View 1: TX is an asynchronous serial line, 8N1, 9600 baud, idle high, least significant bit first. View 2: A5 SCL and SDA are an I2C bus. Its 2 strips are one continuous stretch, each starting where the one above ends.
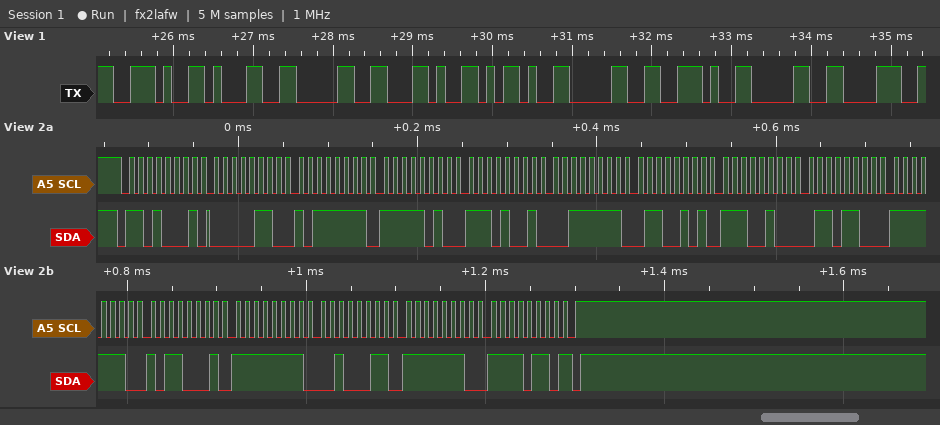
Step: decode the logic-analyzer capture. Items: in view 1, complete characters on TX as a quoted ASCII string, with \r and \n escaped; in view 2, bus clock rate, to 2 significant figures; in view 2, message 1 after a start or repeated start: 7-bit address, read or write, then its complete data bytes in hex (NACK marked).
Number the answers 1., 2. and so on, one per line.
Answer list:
1. ".10,-0.08"
2. 100 kHz
3. 0x68 read: 06 BF FA E9 3F 65 E4 6C FE B1 FF 23 FE F6 NACK
